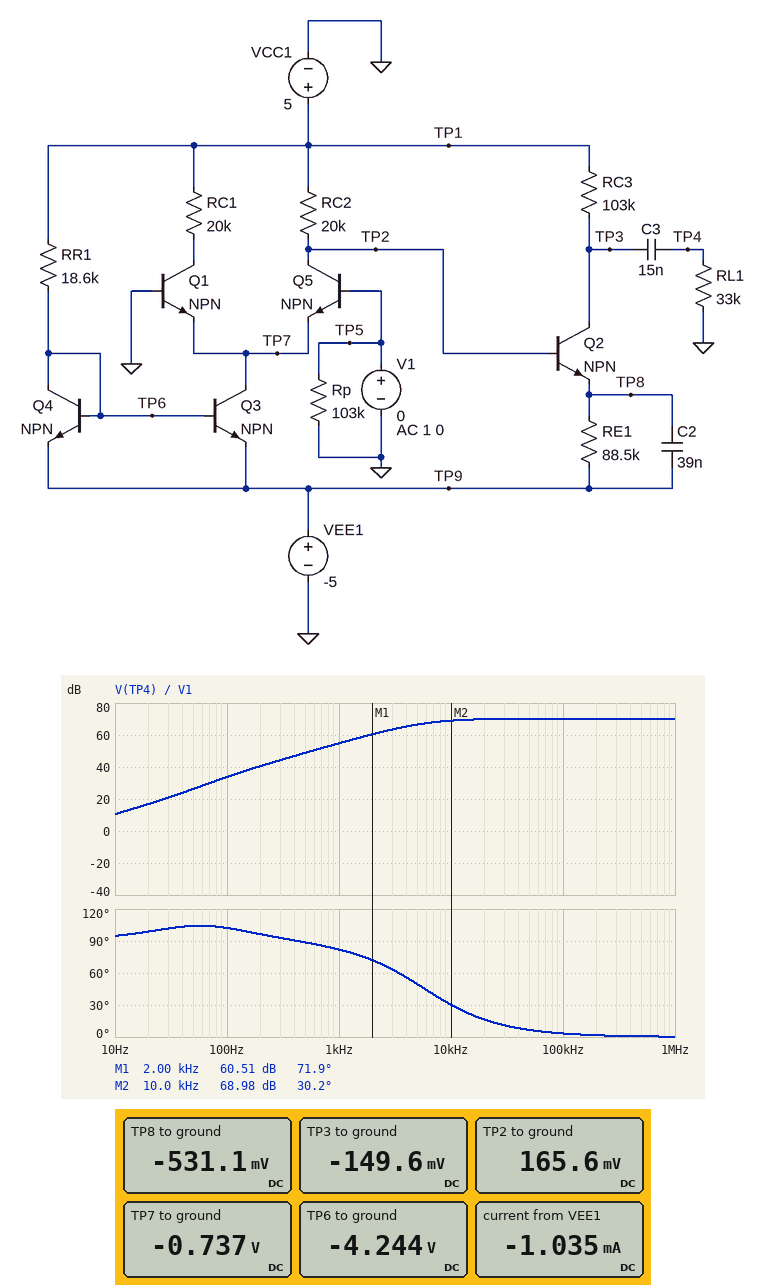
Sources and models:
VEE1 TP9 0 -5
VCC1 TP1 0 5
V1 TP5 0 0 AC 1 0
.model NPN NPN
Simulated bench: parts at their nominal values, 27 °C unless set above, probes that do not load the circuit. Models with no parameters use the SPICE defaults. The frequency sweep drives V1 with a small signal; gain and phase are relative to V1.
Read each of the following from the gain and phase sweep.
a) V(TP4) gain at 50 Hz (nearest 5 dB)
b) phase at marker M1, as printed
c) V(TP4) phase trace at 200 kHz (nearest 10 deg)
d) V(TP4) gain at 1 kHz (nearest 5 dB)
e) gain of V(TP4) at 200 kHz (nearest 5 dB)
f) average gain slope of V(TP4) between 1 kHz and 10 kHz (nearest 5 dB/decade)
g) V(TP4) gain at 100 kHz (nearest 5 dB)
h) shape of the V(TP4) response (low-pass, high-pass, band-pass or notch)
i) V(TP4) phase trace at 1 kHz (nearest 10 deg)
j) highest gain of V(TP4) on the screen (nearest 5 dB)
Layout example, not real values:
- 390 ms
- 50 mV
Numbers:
- 25 dB
- 71.9 deg
- 0 deg
- 55 dB
- 70 dB
- 15 dB/decade
- 70 dB
- high-pass
- 80 deg
- 70 dB
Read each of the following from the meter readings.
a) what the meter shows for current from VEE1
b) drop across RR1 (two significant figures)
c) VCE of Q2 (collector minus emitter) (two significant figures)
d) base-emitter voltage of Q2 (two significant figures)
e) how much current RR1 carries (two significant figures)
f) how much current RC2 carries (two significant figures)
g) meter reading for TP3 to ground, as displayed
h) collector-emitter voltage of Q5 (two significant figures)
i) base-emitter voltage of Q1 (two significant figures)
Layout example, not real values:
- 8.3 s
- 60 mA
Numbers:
- -1.035 mA
- 9.2 V
- 380 mV
- 700 mV
- 500 µA
- 240 µA
- -149.6 mV
- 900 mV
- 740 mV
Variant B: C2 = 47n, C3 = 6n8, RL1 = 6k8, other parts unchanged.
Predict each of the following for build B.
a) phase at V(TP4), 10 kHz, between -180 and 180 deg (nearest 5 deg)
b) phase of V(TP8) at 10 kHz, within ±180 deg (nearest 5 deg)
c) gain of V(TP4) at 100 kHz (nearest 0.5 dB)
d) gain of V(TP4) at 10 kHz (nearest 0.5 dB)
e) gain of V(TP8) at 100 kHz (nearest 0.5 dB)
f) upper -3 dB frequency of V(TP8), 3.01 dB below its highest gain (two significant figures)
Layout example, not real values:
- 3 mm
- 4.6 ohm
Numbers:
- 25 deg
- 115 deg
- 58.5 dB
- 57.5 dB
- 13.0 dB
- 4.8 kHz
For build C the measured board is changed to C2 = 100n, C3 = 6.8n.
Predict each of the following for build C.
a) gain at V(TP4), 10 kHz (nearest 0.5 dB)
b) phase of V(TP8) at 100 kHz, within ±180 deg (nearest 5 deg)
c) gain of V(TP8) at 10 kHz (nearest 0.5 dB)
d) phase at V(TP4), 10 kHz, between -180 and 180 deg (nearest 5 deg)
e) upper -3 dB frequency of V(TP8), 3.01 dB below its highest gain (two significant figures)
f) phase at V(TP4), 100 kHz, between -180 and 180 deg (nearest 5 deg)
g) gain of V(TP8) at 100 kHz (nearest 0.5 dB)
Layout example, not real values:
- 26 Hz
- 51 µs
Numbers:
- 70.0 dB
- 90 deg
- 26.0 dB
- 15 deg
- 2.3 kHz
- 0 deg
- 6.5 dB
